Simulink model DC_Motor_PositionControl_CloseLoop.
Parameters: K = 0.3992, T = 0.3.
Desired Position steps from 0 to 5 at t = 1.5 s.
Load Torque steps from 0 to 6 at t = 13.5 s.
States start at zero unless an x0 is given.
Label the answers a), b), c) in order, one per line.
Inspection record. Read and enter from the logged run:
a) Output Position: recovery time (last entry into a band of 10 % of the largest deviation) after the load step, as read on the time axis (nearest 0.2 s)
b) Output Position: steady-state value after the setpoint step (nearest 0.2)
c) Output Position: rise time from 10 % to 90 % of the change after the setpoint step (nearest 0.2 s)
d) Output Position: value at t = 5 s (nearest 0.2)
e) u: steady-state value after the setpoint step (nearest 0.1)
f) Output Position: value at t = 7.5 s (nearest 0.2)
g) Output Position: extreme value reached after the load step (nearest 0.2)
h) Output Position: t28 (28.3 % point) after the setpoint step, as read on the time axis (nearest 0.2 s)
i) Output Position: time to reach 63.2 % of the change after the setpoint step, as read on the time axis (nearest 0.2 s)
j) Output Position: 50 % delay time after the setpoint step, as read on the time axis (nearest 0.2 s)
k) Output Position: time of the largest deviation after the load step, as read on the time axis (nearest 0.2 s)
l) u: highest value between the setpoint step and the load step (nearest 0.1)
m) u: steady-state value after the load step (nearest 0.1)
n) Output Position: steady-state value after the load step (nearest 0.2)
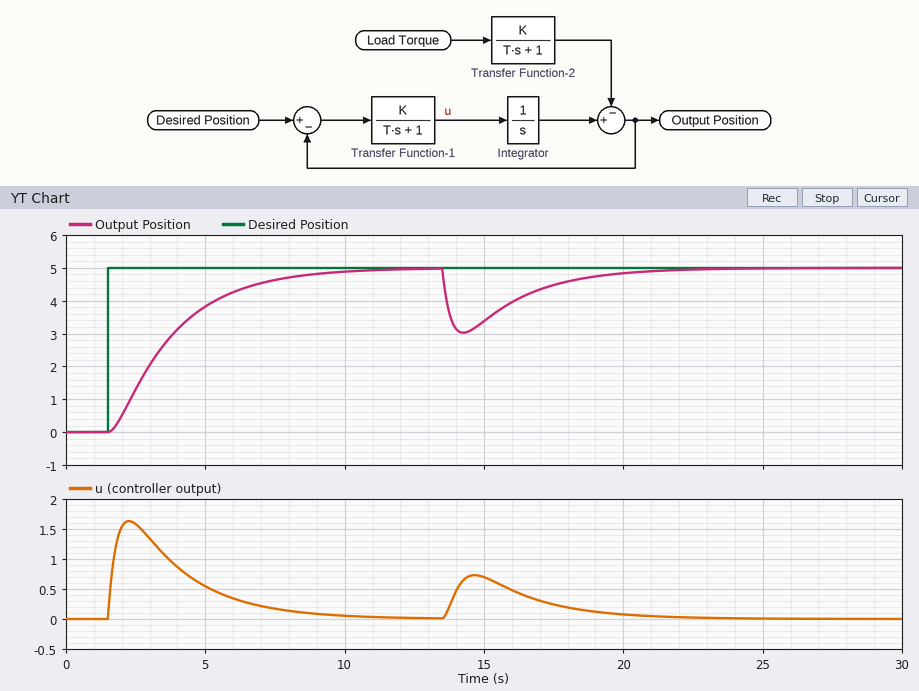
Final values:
a) 19.6 s
b) 5.0
c) 4.8 s
d) 3.8
e) 0.0
f) 4.6
g) 3.0
h) 2.6 s
i) 4.0 s
j) 3.4 s
k) 14.2 s
l) 1.6
m) 0.0
n) 5.0
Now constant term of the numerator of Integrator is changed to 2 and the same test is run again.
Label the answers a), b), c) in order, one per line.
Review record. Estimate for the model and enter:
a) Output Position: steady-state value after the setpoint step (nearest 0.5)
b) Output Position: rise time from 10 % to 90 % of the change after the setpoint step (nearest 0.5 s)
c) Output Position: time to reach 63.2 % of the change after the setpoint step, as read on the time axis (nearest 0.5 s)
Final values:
a) 5.0
b) 2.0 s
c) 3.0 s
